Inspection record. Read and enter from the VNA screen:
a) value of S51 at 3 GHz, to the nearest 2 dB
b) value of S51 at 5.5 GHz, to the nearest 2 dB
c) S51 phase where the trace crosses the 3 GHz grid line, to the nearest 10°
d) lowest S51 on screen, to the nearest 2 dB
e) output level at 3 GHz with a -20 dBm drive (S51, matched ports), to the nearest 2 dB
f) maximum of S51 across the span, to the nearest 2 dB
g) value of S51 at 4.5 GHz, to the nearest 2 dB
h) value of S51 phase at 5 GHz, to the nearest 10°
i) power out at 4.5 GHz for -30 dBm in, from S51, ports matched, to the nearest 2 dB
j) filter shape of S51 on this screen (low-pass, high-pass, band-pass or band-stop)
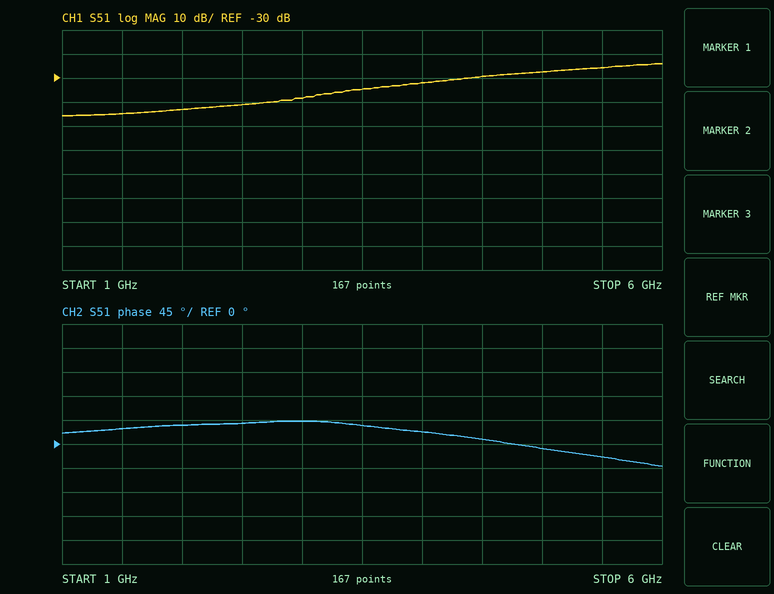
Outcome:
-38 dB
-26 dB
40°
-46 dB
-58 dBm
-24 dB
-30 dB
-10°
-60 dBm
high-pass
